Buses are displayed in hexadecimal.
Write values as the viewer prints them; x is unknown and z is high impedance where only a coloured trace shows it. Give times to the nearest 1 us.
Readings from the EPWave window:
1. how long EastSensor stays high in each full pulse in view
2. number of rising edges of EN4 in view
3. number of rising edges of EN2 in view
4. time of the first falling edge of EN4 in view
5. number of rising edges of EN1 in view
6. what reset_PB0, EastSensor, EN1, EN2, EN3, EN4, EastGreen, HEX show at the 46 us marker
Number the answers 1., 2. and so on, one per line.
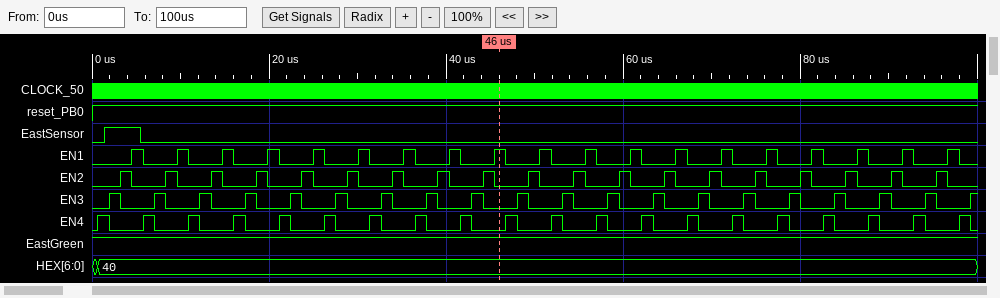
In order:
1. 4 us
2. 20
3. 19
4. 2 us
5. 19
6. reset_PB0=1, EastSensor=0, EN1=1, EN2=0, EN3=0, EN4=0, EastGreen=1, HEX=40
